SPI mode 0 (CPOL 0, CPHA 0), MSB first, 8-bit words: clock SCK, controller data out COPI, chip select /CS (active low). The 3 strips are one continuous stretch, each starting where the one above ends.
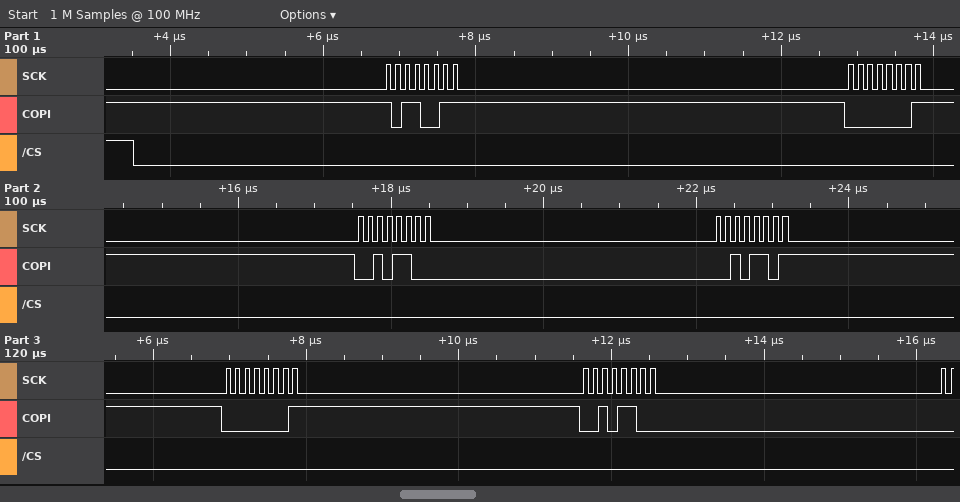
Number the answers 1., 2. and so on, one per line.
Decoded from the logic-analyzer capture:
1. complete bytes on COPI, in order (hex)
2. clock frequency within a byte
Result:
1. B3 01 2C 2D 01 2C
2. 8 MHz
